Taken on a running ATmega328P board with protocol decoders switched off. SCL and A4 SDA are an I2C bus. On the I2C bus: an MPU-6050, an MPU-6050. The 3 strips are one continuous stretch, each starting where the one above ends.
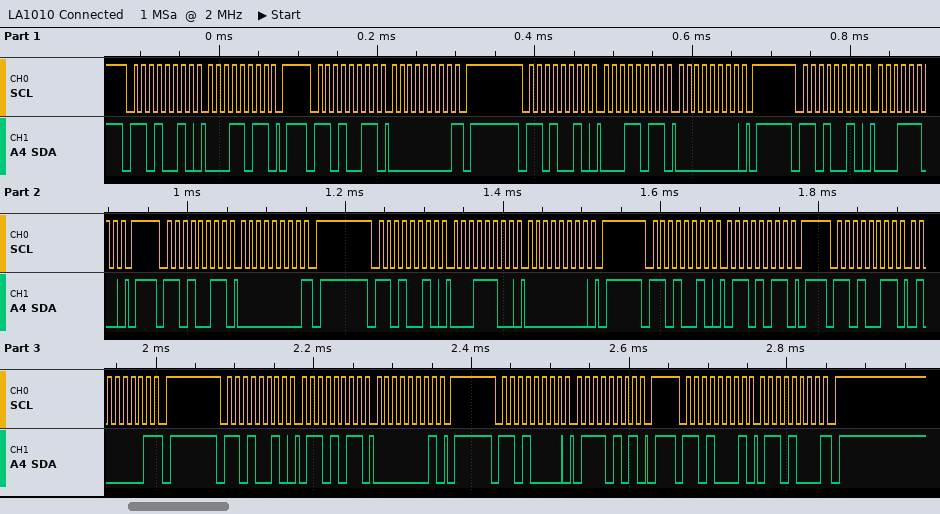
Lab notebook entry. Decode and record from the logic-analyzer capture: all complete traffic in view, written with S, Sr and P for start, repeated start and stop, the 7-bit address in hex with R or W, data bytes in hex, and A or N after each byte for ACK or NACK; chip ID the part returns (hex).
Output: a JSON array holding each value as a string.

["S 69W A 1B A P S 69R A 00 N P S 69W A 1B A 00 A P S 69W A 1C A P S 69R A 00 N P S 69W A 1C A 00 A P S 69W A 6B A P S 69R A 41 N P S 69W A 6B A 01 A P S 68W A 75 A P S 68R A 68 N P", "0x68"]
